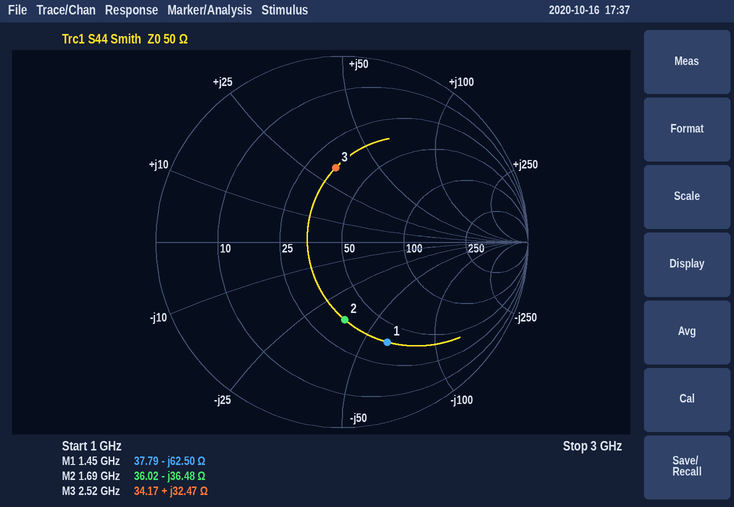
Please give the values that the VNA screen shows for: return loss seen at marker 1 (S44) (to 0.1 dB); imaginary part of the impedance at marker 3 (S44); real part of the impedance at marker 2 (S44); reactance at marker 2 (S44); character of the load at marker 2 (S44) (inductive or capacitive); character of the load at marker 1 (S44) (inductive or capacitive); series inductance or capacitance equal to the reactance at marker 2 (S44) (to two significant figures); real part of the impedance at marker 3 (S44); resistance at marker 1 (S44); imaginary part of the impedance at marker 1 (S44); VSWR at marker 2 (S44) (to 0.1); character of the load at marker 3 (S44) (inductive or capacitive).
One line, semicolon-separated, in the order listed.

4.6 dB; +32.47 Ω; 36.02 Ω; -36.48 Ω; capacitive; capacitive; 2.6 pF; 34.17 Ω; 37.79 Ω; -62.50 Ω; 2.4; inductive
